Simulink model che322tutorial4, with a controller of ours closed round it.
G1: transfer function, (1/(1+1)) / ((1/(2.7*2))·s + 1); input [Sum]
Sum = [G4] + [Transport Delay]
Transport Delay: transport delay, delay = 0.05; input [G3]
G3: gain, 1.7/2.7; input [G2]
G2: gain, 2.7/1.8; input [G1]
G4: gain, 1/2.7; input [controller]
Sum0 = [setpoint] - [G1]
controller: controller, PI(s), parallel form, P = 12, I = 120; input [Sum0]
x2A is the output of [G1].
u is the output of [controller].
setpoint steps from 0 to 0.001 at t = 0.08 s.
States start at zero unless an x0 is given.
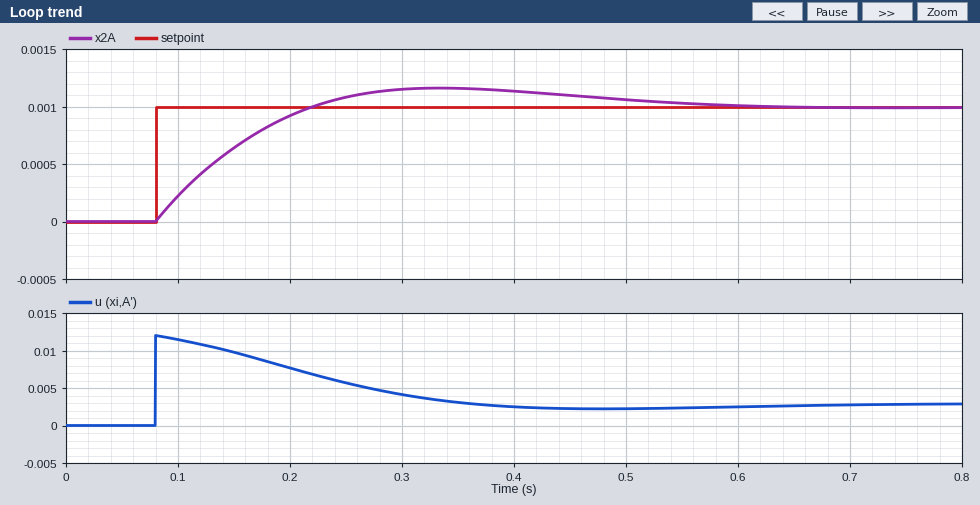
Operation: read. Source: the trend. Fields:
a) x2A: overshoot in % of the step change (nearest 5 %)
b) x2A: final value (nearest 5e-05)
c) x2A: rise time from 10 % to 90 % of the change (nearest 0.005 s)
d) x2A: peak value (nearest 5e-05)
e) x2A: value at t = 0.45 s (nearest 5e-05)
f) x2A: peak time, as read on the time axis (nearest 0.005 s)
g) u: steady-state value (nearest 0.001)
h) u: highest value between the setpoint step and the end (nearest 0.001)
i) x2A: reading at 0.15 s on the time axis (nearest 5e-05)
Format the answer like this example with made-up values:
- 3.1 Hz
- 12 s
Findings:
- 15 %
- 0.00100
- 0.105 s
- 0.00115
- 0.00110
- 0.335 s
- 0.003
- 0.012
- 0.00065
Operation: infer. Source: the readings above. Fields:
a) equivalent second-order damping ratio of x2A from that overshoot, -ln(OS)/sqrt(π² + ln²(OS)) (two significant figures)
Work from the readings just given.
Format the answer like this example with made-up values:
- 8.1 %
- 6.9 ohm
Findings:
- 0.52
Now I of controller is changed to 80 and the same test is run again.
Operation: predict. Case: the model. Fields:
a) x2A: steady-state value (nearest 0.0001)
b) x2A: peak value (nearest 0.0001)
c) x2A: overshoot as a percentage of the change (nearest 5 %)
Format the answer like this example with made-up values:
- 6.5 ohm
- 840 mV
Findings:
- 0.0010
- 0.0011
- 10 %
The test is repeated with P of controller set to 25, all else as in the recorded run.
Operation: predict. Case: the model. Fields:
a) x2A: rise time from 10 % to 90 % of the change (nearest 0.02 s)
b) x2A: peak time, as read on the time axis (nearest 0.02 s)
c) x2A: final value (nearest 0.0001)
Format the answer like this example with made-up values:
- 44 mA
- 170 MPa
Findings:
- 0.08 s
- 0.30 s
- 0.0010
